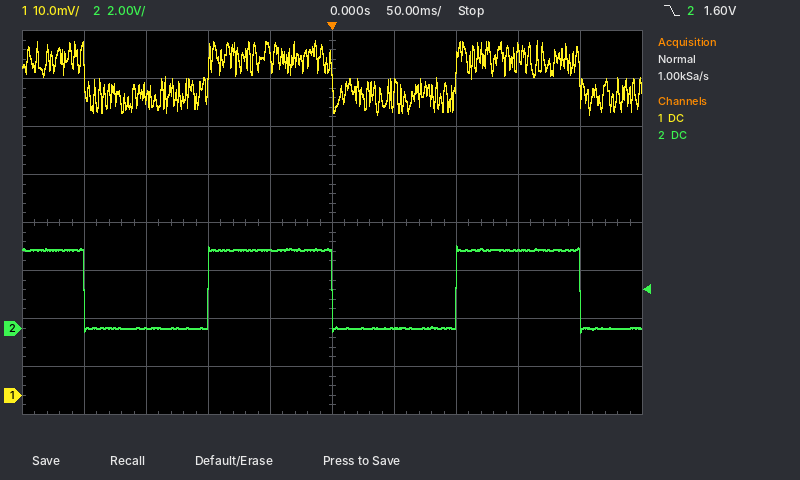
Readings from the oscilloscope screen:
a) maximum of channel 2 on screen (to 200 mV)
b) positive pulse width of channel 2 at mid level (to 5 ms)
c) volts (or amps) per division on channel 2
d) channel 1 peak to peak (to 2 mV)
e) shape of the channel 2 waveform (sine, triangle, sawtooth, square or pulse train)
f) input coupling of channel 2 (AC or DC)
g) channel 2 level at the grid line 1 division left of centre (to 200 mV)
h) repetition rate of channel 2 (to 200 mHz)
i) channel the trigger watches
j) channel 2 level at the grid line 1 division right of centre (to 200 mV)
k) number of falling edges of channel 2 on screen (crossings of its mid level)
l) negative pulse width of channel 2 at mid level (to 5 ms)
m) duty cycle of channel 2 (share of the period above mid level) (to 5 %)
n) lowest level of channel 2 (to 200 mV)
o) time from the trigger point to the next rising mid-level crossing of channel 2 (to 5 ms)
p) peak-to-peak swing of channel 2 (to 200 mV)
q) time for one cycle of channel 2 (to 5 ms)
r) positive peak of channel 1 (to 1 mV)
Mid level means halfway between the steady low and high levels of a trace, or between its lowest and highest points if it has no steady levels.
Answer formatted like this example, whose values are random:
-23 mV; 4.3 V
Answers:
3.4 V; 100 ms; 2 V; 16 mV; square; DC; 3.2 V; 5.0 Hz; channel 2; 0.0 V; 3; 100 ms; 50 %; -200 mV; 100 ms; 3.6 V; 200 ms; 74 mV
